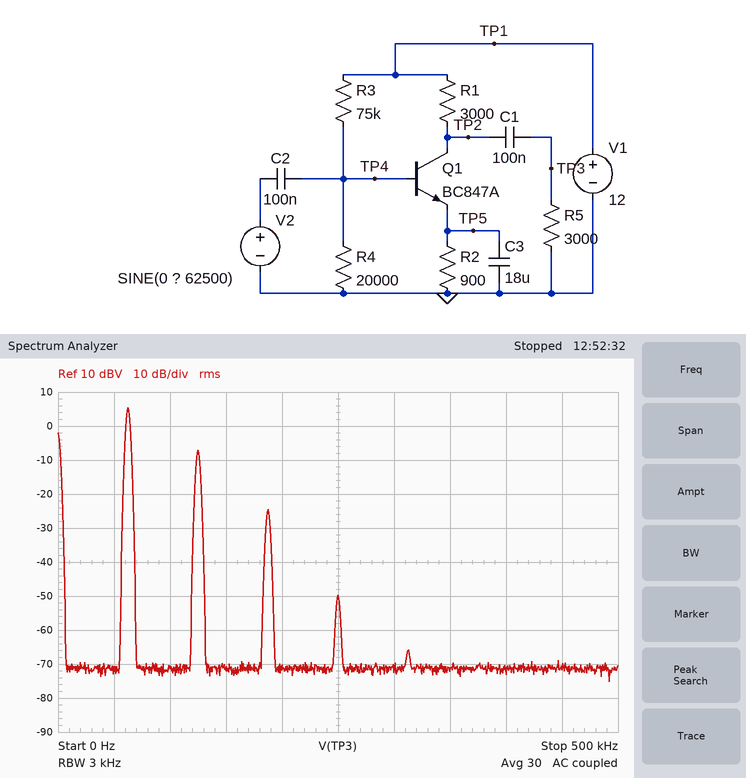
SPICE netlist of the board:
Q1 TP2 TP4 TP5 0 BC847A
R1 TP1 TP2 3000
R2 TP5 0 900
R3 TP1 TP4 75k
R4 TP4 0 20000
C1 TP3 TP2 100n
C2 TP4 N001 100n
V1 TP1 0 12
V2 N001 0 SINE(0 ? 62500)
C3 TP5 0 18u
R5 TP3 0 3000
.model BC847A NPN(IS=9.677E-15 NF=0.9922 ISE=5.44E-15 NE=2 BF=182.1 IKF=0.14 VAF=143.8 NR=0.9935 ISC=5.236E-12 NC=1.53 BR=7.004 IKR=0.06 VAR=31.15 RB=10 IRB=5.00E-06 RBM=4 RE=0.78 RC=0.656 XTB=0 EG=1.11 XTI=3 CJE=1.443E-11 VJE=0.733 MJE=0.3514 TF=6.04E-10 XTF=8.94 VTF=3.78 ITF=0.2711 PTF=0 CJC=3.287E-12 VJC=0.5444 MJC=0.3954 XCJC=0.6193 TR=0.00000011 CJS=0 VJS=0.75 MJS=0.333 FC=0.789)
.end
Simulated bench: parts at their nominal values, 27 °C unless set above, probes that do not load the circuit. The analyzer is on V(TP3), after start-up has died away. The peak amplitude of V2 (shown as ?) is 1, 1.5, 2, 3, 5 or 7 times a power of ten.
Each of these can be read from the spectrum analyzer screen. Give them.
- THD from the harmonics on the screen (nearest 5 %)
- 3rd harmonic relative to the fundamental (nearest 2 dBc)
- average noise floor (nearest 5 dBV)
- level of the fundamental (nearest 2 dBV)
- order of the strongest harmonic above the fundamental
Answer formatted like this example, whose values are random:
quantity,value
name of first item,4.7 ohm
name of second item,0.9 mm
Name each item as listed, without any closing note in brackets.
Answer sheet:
quantity,value
THD from the harmonics on the screen,25 %
3rd harmonic relative to the fundamental,-30 dBc
average noise floor,-70 dBV
level of the fundamental,6 dBV
order of the strongest harmonic above the fundamental,2
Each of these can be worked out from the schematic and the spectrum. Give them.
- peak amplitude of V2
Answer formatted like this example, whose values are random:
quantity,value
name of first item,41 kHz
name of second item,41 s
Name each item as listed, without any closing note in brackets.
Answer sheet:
quantity,value
peak amplitude of V2,30 mV
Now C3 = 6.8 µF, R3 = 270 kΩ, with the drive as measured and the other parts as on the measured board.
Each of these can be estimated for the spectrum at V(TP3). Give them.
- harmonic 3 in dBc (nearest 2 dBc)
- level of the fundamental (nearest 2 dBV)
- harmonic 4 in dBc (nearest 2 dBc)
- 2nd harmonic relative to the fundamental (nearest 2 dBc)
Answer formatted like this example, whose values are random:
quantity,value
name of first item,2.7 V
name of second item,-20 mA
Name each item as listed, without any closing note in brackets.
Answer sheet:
quantity,value
harmonic 3 in dBc,-26 dBc
level of the fundamental,-12 dBV
harmonic 4 in dBc,-44 dBc
2nd harmonic relative to the fundamental,-12 dBc
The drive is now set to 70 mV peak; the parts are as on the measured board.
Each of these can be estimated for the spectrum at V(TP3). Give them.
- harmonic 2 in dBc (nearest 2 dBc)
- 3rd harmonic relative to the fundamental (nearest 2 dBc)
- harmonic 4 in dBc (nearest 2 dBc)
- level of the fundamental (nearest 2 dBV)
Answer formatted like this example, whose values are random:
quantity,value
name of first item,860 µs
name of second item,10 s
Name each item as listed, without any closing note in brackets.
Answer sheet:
quantity,value
harmonic 2 in dBc,-6 dBc
3rd harmonic relative to the fundamental,-18 dBc
harmonic 4 in dBc,-46 dBc
level of the fundamental,8 dBV
